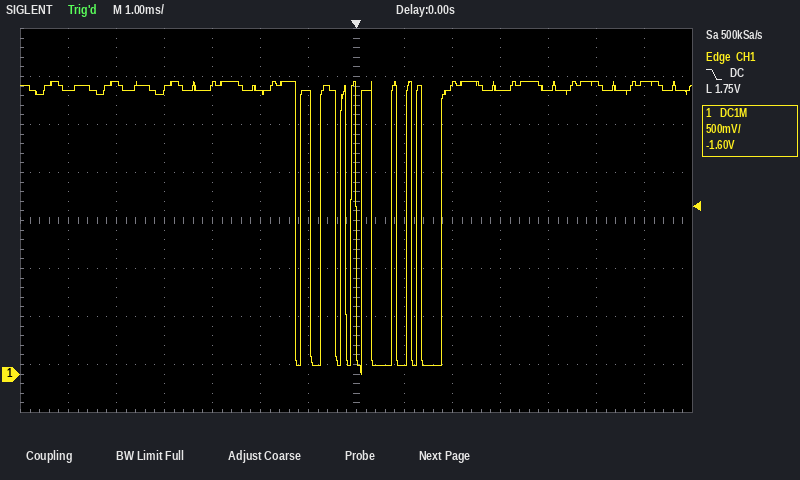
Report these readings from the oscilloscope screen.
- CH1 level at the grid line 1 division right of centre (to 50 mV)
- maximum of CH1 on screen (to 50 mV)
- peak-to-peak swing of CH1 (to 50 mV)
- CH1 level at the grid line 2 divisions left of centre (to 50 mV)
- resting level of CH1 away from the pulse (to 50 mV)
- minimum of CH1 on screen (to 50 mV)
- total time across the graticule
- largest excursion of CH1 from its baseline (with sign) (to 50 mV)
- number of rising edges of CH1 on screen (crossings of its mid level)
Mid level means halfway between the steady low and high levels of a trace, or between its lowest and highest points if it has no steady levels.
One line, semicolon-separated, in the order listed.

100 mV; 3.05 V; 3.05 V; 2.95 V; 2.95 V; 0 mV; 14 ms; -2.95 V; 9
